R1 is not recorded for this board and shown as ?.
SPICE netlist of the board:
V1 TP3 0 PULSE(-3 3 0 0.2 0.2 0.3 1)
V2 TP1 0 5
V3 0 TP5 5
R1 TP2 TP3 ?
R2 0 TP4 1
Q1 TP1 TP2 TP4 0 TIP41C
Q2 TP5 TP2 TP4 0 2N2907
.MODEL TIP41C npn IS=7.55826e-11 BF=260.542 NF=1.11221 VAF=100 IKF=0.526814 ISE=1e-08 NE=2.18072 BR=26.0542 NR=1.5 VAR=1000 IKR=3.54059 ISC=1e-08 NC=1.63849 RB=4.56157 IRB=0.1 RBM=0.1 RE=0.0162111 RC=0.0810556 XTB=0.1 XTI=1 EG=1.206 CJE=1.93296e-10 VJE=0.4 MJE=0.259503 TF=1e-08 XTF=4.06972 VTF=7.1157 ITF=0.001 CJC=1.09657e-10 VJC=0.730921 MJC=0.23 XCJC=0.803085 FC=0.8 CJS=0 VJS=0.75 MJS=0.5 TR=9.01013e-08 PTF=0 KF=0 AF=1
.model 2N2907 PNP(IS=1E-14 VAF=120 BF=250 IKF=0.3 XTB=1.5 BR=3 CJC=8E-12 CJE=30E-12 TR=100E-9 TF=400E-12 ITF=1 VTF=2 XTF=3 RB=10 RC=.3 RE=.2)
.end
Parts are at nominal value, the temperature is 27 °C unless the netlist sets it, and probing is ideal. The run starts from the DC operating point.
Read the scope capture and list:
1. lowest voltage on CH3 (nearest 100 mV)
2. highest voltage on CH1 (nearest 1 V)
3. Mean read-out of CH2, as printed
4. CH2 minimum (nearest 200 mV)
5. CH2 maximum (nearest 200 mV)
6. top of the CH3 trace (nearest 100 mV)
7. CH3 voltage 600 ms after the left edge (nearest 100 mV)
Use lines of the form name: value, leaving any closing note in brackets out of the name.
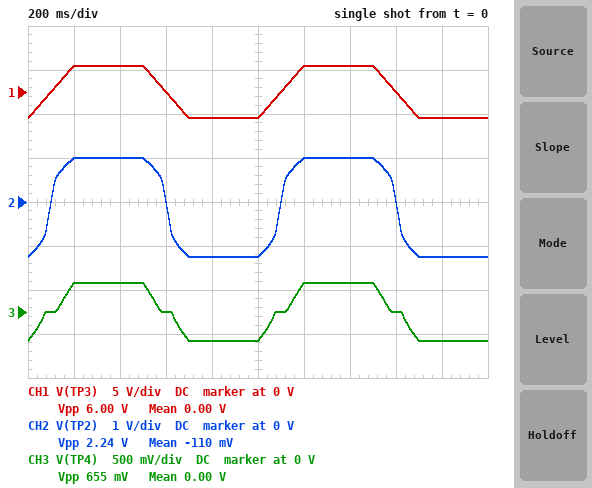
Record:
lowest voltage on CH3: -300 mV
highest voltage on CH1: 3 V
Mean read-out of CH2, as printed: -110 mV
CH2 minimum: -1.2 V
CH2 maximum: 1.0 V
top of the CH3 trace: 300 mV
CH3 voltage 600 ms after the left edge: 0 V
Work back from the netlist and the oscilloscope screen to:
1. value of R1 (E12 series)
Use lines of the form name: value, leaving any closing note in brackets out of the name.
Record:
value of R1: 680 Ω
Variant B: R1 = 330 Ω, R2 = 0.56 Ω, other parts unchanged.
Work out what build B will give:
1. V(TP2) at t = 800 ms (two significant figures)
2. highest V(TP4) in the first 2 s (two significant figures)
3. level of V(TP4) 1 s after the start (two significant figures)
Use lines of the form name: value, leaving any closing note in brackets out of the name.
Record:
V(TP2) at t = 800 ms: -1.3 V
highest V(TP4) in the first 2 s: 330 mV
level of V(TP4) 1 s after the start: -290 mV
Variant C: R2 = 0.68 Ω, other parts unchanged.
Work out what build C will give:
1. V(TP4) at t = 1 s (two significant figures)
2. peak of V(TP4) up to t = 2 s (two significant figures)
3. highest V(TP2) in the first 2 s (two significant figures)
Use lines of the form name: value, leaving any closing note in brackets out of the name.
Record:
V(TP4) at t = 1 s: -230 mV
peak of V(TP4) up to t = 2 s: 230 mV
highest V(TP2) in the first 2 s: 900 mV
